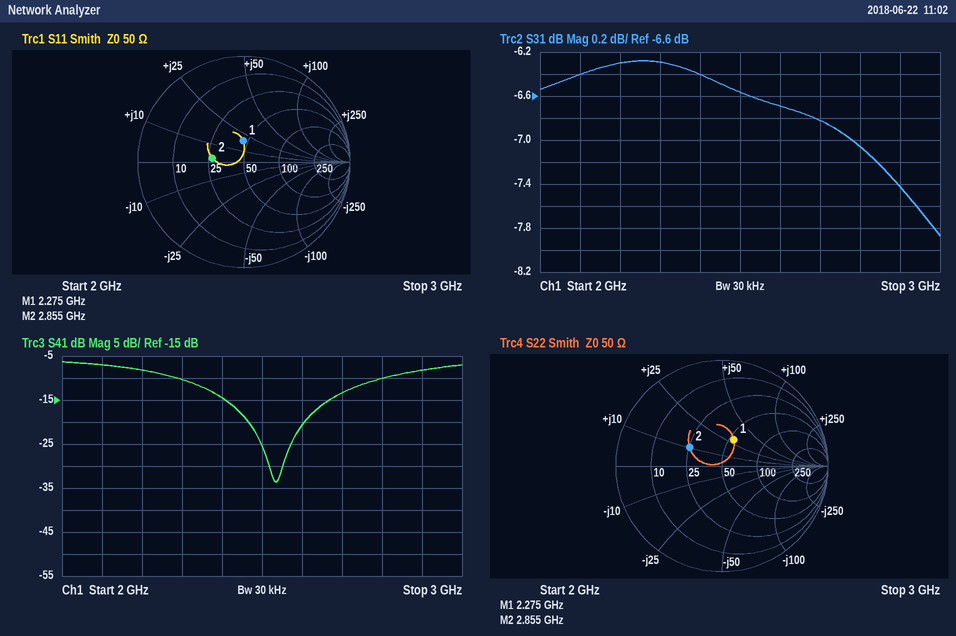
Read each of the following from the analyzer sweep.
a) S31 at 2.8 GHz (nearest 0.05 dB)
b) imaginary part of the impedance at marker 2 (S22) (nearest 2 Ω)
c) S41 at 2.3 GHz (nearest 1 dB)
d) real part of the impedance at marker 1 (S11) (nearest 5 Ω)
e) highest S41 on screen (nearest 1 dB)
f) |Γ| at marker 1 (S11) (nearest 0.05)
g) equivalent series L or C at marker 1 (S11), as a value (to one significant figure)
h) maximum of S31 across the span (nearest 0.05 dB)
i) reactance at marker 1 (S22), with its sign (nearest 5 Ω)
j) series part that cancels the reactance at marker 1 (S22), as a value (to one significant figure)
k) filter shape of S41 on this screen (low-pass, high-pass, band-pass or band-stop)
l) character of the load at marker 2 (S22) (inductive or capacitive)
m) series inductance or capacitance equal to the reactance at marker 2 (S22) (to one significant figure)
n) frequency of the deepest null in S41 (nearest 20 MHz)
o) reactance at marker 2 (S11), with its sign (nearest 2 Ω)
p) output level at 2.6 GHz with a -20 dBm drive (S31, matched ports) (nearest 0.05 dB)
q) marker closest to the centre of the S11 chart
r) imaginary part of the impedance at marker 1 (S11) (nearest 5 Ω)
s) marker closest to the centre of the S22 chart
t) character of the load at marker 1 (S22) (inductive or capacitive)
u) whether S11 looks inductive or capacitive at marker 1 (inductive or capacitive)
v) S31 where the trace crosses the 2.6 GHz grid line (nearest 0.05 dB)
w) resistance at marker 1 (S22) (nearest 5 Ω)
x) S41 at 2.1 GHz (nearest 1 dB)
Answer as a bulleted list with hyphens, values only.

- -7.05 dB
- +10 Ω
- -10 dB
- 45 Ω
- -6 dB
- 0.20
- 1 nH
- -6.30 dB
- +30 Ω
- 2 pF
- band-stop
- inductive
- 600 pH
- 2.54 GHz
- +2 Ω
- -26.70 dBm
- marker 1
- +20 Ω
- marker 1
- inductive
- inductive
- -6.70 dB
- 55 Ω
- -7 dB
